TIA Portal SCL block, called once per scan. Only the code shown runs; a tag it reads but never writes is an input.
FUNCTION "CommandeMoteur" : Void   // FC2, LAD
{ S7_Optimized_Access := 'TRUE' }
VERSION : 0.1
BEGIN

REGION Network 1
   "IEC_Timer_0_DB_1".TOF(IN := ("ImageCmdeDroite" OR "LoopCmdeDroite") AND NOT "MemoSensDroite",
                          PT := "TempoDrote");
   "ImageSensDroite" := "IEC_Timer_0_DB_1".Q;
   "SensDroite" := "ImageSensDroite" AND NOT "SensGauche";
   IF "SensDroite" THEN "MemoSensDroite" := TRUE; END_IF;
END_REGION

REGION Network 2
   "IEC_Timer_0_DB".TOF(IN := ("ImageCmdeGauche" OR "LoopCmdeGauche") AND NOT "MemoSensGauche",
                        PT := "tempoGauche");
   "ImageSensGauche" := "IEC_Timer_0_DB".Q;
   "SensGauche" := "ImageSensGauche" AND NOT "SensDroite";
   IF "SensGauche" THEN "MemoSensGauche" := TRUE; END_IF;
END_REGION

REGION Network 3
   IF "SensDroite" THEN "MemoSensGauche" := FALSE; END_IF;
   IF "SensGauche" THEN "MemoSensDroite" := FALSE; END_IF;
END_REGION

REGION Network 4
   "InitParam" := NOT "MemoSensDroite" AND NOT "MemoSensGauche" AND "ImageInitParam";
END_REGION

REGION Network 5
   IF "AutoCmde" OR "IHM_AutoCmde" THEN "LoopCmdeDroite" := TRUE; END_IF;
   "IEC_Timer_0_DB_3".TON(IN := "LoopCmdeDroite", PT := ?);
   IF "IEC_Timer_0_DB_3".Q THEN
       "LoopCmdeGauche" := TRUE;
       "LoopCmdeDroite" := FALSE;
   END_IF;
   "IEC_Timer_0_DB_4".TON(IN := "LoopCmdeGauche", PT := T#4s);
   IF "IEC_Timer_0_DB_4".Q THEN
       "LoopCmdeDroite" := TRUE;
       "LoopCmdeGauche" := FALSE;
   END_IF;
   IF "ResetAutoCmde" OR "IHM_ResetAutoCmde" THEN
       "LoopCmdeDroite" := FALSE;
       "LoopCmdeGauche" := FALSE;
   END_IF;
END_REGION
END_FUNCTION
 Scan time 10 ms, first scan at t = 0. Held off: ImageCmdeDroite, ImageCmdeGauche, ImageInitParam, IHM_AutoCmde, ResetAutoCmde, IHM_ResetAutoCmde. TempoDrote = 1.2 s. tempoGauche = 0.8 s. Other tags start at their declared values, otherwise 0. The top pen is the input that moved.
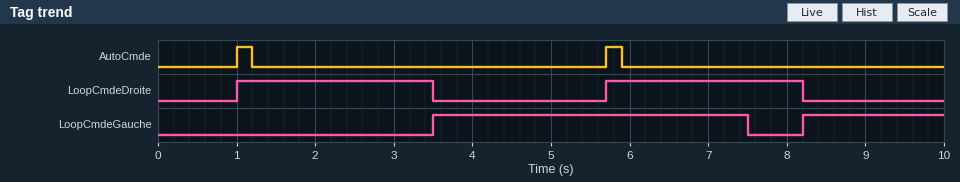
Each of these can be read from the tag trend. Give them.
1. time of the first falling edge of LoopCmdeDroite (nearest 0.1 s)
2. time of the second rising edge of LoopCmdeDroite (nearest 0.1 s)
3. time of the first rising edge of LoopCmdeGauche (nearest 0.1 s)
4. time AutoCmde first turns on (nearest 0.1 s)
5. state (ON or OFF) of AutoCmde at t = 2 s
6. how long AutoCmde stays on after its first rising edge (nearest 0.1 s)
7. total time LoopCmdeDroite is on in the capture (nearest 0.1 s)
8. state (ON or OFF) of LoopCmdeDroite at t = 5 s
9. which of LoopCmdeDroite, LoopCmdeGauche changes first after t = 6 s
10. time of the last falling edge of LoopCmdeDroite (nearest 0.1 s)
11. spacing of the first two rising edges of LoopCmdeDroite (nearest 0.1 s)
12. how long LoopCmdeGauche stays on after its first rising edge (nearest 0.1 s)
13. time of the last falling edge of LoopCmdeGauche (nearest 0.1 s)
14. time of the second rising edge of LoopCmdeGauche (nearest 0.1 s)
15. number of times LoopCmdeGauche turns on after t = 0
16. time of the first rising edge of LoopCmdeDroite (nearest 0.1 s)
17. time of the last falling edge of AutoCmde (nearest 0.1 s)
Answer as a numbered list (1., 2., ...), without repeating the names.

1. 3.5 s
2. 5.7 s
3. 3.5 s
4. 1.0 s
5. OFF
6. 0.2 s
7. 5.0 s
8. OFF
9. LoopCmdeGauche
10. 8.2 s
11. 4.7 s
12. 4.0 s
13. 7.5 s
14. 8.2 s
15. 2
16. 1.0 s
17. 5.9 s
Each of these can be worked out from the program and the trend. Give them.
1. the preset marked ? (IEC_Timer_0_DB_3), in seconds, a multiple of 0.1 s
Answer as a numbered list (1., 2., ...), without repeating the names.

1. 2.5 s
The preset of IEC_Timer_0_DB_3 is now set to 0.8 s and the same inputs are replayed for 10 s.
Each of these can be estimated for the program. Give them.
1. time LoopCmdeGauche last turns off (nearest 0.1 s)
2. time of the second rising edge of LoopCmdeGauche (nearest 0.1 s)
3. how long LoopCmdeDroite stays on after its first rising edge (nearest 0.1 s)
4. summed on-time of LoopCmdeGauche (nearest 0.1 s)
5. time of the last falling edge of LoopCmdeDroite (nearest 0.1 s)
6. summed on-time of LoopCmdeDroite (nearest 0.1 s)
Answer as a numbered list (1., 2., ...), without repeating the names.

1. 5.8 s
2. 6.5 s
3. 0.8 s
4. 7.5 s
5. 6.5 s
6. 1.6 s
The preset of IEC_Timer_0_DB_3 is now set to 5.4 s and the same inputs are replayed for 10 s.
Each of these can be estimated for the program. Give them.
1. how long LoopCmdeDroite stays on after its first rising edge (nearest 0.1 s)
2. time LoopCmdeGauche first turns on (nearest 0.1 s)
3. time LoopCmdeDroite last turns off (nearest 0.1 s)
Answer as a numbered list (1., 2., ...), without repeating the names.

1. 5.4 s
2. 6.4 s
3. 6.4 s
